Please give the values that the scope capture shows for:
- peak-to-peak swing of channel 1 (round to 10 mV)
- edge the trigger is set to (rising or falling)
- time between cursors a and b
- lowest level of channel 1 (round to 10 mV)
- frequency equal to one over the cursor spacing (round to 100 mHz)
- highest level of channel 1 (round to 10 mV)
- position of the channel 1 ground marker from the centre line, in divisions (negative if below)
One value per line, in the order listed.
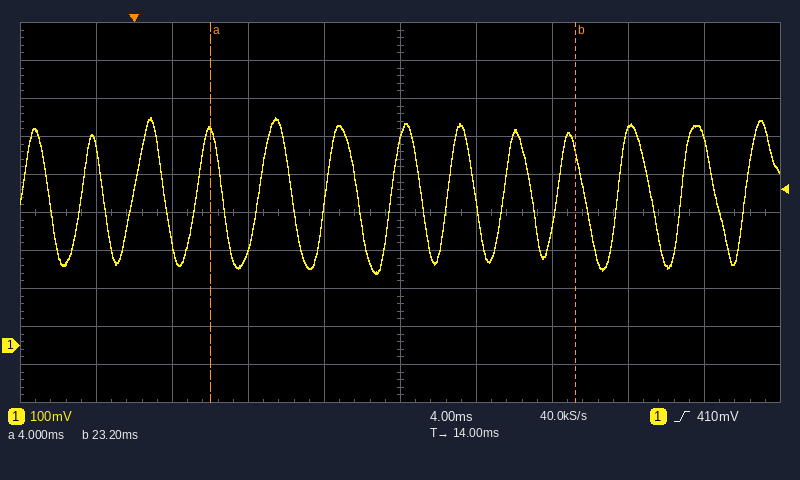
410 mV
rising
19.2 ms
190 mV
52.1 Hz
600 mV
-3.5 div
